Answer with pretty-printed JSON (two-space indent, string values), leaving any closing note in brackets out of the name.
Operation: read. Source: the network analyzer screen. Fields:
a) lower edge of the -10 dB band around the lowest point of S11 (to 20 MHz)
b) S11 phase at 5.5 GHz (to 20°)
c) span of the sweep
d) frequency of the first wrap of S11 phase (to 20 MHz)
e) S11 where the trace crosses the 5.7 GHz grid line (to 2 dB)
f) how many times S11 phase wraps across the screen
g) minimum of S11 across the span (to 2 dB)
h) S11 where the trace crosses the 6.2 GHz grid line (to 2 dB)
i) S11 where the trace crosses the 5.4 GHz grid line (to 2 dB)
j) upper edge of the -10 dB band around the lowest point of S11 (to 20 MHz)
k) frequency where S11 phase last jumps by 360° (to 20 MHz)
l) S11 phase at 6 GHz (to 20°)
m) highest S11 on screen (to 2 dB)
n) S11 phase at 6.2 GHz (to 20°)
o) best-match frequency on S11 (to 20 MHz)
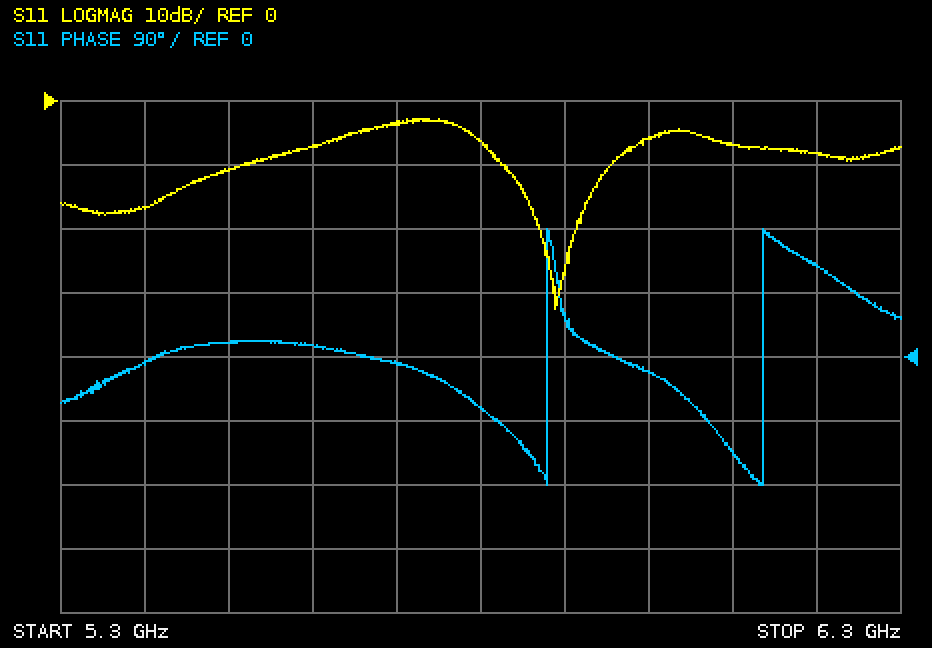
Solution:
{
  "lower edge of the -10 dB band around the lowest point of S11": "5.82 GHz",
  "S11 phase at 5.5 GHz": "20°",
  "span of the sweep": "1 GHz",
  "frequency of the first wrap of S11 phase": "5.88 GHz",
  "S11 where the trace crosses the 5.7 GHz grid line": "-4 dB",
  "how many times S11 phase wraps across the screen": "2",
  "minimum of S11 across the span": "-32 dB",
  "S11 where the trace crosses the 6.2 GHz grid line": "-8 dB",
  "S11 where the trace crosses the 5.4 GHz grid line": "-16 dB",
  "upper edge of the -10 dB band around the lowest point of S11": "5.96 GHz",
  "frequency where S11 phase last jumps by 360°": "6.14 GHz",
  "S11 phase at 6 GHz": "-20°",
  "highest S11 on screen": "-2 dB",
  "S11 phase at 6.2 GHz": "120°",
  "best-match frequency on S11": "5.88 GHz"
}
